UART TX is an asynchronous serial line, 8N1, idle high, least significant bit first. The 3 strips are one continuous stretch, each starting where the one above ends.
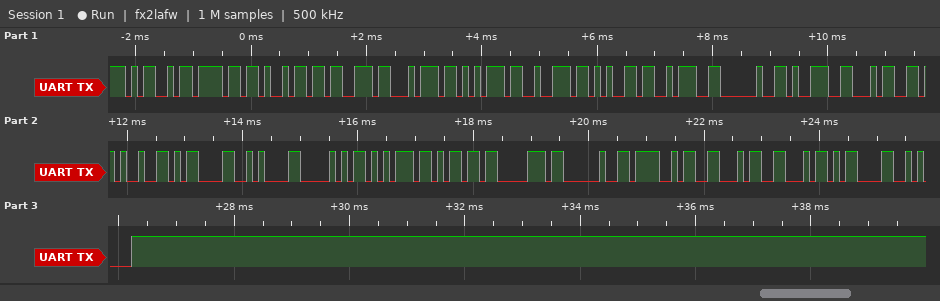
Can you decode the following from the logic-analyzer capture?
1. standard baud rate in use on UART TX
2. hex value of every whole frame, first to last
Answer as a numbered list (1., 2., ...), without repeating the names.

1. 9600 baud
2. 4D 6F 69 73 74 75 72 65 3A 20 39 34 25 0D 0A 50 75 6D 70 20 4F 46 46 0D 0A
